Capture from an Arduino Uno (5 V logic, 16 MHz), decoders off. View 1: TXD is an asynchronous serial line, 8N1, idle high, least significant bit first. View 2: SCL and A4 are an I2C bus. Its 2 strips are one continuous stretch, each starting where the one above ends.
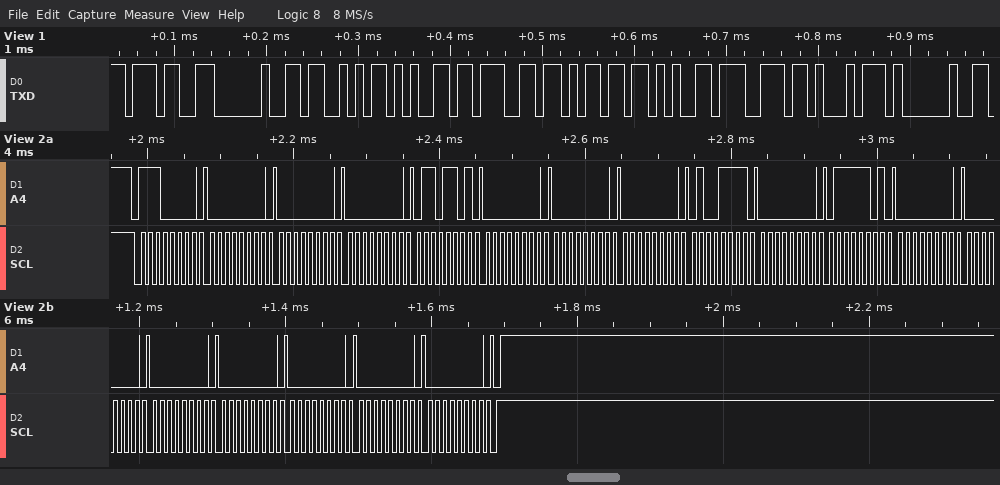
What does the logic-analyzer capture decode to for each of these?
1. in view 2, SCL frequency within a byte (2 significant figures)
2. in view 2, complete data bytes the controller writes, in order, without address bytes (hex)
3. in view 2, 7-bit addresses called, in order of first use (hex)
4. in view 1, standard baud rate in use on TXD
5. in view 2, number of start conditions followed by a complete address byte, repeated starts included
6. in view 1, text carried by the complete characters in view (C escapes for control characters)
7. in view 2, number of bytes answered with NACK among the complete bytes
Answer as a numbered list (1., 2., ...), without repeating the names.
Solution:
1. 100 kHz
2. 00 00 00 6D 00 00 00 4F 00 7D 00 00 00 00 00 00 00
3. 0x70
4. 115200 baud
5. 1
6. "7 Segment "
7. 0
